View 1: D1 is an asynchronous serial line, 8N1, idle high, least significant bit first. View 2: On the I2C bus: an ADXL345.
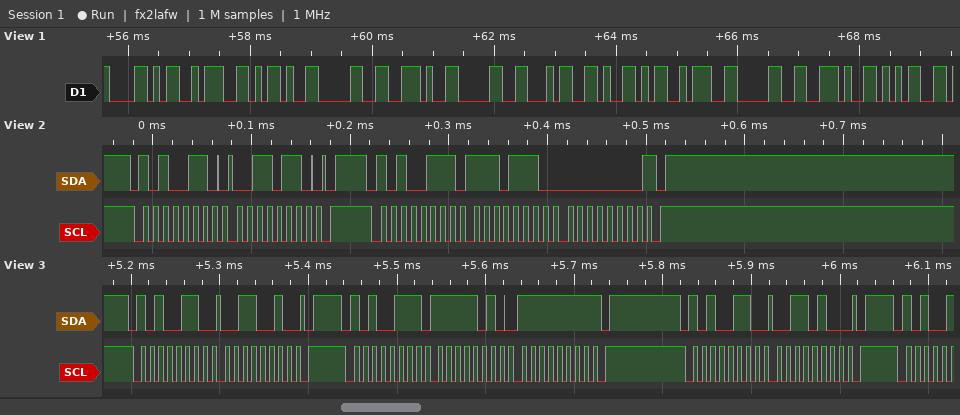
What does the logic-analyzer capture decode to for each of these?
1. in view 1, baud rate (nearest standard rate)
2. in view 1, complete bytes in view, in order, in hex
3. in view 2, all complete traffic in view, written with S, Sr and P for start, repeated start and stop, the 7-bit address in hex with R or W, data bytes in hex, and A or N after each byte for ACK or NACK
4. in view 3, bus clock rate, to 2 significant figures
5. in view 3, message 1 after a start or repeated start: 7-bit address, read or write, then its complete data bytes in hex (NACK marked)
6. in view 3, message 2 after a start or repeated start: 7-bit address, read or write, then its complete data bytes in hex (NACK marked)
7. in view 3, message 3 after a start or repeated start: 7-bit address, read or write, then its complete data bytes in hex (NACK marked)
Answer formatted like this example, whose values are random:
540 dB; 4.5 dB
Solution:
9600 baud; 58 3A 2D 30 2E 30 34 59 3A 30 2E 35; S 53W A 36 A P S 53R A EE A 00 N P; 100 kHz; 0x53 write: 32; 0x53 read: FA FF NACK; 0x53 write: 34
